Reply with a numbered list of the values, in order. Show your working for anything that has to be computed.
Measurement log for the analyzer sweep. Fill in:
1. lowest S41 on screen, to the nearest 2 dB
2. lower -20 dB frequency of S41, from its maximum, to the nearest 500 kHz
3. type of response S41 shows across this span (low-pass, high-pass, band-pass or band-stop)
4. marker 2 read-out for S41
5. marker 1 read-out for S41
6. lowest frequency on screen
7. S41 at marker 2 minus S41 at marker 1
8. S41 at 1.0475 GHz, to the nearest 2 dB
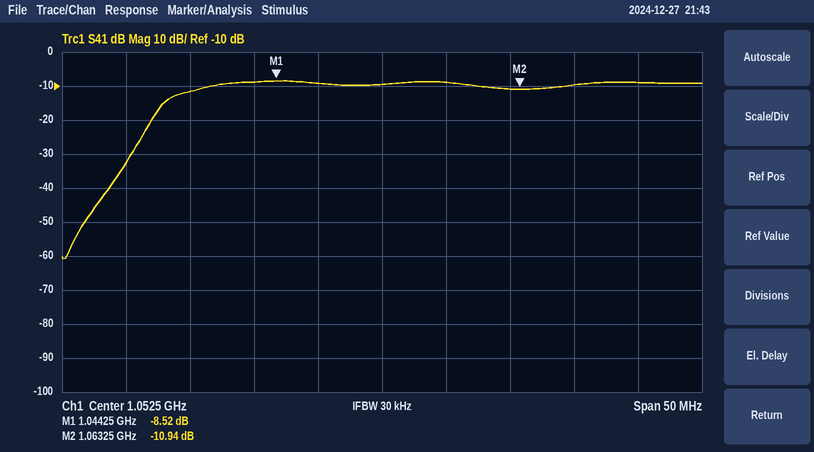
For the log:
1. -60 dB
2. 1.0330 GHz
3. high-pass
4. -10.94 dB
5. -8.52 dB
6. 1.0275 GHz
7. -10.94 − (-8.52) = -2.42 dB
8. -10 dB
